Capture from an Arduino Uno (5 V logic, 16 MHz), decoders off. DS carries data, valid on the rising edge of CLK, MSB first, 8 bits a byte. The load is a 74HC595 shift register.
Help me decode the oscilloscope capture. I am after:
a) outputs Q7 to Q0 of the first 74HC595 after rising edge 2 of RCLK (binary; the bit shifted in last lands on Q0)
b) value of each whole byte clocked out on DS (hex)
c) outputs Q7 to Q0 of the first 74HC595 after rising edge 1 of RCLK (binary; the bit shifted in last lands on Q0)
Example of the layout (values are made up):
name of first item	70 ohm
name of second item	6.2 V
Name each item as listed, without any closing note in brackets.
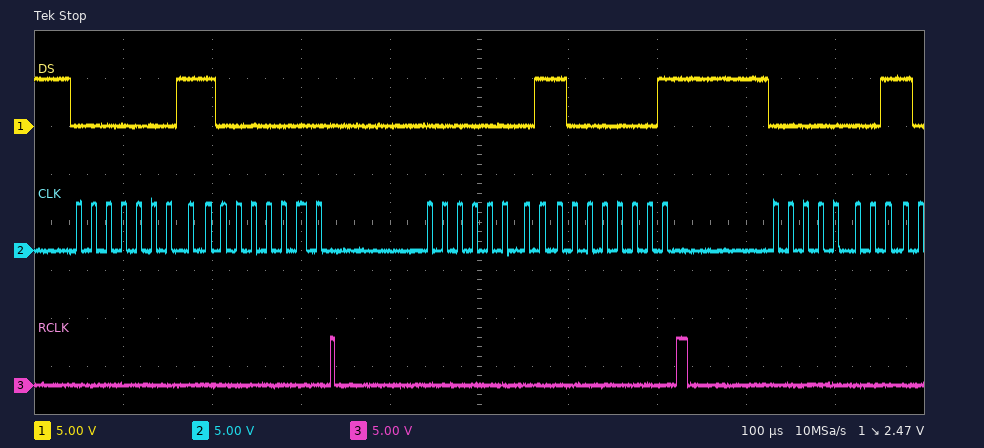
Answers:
outputs Q7 to Q0 of the first 74HC595 after rising edge 2 of RCLK	10000001
value of each whole byte clocked out on DS	01 80 01 81 01
outputs Q7 to Q0 of the first 74HC595 after rising edge 1 of RCLK	10000000
